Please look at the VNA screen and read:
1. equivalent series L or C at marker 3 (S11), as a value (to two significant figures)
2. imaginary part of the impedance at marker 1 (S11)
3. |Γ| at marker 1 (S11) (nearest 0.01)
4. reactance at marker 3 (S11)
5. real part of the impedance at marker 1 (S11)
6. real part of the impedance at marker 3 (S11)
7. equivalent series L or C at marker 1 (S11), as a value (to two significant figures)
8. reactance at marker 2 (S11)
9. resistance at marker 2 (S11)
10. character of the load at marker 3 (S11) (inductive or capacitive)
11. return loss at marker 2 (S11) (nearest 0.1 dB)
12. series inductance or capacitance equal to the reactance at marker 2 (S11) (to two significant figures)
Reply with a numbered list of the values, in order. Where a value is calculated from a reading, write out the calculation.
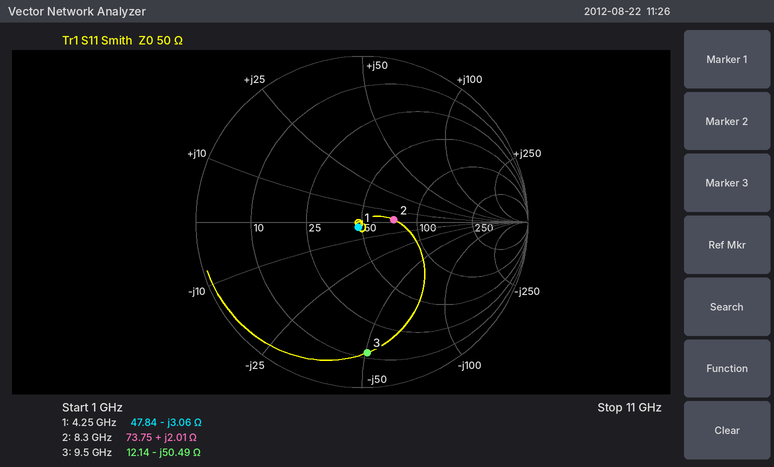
1. C = 1/(2π × 9.5 GHz × 50.49 Ω) ≈ 332 fF, so 330 fF to two significant figures
2. -3.06 Ω
3. 0.04
4. -50.49 Ω
5. 47.84 Ω
6. 12.14 Ω
7. C = 1/(2π × 4.25 GHz × 3.06 Ω) ≈ 12 pF
8. +2.01 Ω
9. 73.75 Ω
10. capacitive
11. 14.3 dB
12. L = 2.01 Ω/(2π × 8.3 GHz) ≈ 39 pH
